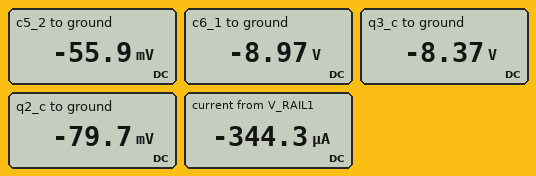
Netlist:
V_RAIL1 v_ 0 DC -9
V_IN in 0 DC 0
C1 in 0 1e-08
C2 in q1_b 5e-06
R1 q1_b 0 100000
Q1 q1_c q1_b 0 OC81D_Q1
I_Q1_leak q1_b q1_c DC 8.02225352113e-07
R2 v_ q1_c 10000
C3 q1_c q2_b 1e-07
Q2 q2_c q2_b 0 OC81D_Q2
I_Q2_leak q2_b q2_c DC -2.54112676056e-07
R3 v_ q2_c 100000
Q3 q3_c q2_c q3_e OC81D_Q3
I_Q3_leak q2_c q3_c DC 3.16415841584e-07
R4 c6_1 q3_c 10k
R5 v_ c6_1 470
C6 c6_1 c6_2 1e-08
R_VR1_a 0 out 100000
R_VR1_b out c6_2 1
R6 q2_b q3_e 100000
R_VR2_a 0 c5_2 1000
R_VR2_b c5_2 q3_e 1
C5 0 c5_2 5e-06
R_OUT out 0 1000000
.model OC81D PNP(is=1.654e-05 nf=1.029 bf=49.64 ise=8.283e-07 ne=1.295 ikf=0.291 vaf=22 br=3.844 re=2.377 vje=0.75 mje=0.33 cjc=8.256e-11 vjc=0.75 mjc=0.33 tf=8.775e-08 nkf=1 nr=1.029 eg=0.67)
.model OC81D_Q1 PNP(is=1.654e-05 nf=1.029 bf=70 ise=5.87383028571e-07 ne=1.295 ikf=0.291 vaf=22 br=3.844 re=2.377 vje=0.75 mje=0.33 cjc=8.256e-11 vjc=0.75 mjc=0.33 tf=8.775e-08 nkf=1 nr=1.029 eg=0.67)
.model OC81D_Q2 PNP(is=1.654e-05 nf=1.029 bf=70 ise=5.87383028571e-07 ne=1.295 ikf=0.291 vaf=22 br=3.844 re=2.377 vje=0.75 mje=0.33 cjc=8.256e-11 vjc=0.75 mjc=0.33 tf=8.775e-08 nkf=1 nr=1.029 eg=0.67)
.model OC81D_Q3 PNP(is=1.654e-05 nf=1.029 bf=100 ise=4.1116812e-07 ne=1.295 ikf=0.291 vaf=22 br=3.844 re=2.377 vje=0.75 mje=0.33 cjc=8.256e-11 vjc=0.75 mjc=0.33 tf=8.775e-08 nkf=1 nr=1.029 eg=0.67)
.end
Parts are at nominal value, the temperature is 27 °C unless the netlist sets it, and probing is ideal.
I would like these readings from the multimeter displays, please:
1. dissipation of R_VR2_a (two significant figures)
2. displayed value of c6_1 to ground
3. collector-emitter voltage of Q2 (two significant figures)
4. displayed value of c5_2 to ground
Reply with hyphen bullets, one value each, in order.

- 3.1 µW
- -8.97 V
- -80 mV
- -55.9 mV
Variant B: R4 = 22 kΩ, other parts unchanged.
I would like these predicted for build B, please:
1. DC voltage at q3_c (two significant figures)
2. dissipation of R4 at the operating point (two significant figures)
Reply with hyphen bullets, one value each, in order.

- -7.7 V
- 78 µW
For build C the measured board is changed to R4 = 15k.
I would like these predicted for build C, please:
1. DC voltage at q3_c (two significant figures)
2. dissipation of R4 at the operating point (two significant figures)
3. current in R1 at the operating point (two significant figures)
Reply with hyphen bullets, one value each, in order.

- -8.1 V
- 54 µW
- 580 nA
